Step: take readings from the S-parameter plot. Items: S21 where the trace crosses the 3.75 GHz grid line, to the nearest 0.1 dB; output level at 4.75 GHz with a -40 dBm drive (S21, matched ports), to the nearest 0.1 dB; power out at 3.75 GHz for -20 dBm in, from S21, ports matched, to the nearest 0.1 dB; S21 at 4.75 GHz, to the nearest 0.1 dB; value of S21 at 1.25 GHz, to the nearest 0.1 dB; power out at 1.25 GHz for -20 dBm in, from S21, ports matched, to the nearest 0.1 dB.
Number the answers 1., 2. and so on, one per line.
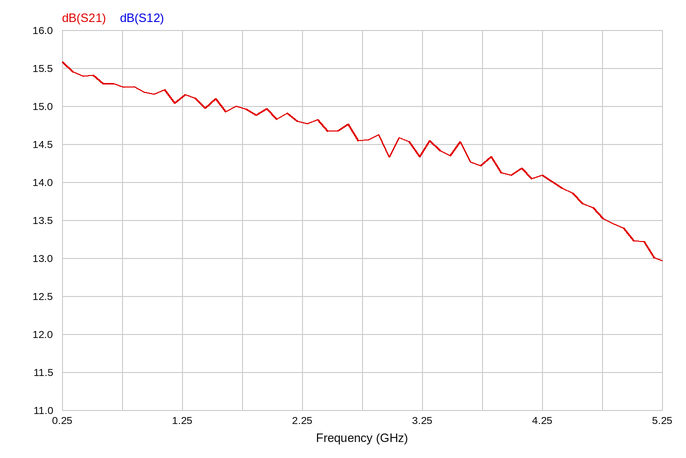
1. 14.2 dB
2. -26.5 dBm
3. -5.8 dBm
4. 13.5 dB
5. 15.1 dB
6. -4.9 dBm
